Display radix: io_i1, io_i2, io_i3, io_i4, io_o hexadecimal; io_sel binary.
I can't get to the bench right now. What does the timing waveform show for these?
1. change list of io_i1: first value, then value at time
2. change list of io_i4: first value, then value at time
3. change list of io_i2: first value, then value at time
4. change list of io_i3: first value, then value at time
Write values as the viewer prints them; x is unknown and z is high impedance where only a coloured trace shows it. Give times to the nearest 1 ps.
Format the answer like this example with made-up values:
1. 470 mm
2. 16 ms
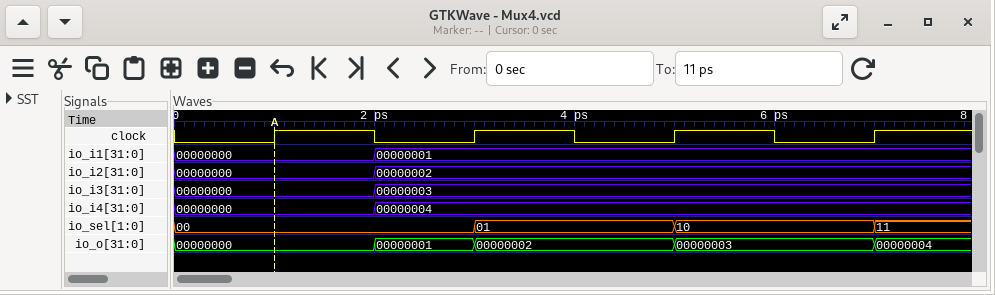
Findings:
1. 00000000, 00000001 at 2 ps
2. 00000000, 00000004 at 2 ps
3. 00000000, 00000002 at 2 ps
4. 00000000, 00000003 at 2 ps
